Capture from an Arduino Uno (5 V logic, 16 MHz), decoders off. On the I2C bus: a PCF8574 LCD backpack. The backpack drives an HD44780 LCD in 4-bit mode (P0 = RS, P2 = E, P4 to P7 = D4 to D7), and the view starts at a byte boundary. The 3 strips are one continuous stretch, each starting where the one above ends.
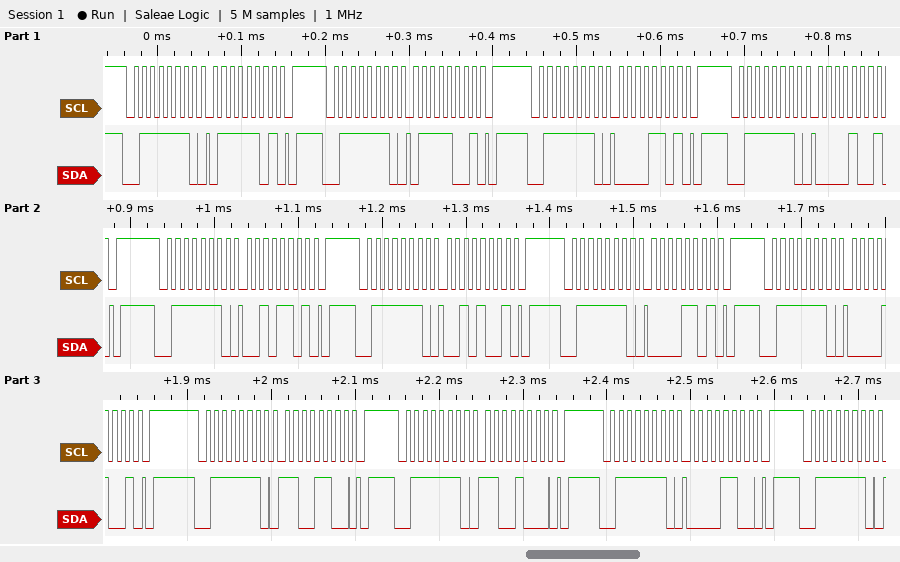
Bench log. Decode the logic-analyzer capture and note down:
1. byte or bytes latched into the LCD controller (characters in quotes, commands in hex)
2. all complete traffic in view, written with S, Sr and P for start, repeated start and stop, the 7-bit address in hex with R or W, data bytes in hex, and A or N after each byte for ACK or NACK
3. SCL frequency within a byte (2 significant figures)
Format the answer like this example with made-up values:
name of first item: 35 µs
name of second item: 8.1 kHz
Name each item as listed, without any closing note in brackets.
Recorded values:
byte or bytes latched into the LCD controller: 'p' ' '
all complete traffic in view, written with S, Sr and P for start, repeated start and stop, the 7-bit address in hex with R or W, data bytes in hex, and A or N after each byte for ACK or NACK: S 3FW A 7D A P S 3FW A 79 A P S 3FW A 0D A P S 3FW A 09 A P S 3FW A 2D A P S 3FW A 29 A P S 3FW A 0D A P S 3FW A 09 A P S 3FW A CC A P S 3FW A C8 A P S 3FW A 0C A P S 3FW A
SCL frequency within a byte: 100 kHz
